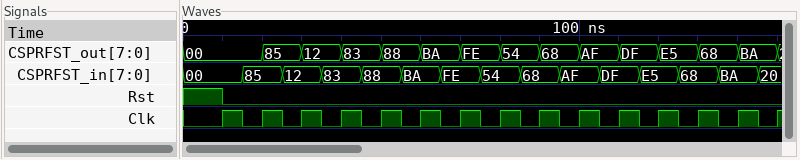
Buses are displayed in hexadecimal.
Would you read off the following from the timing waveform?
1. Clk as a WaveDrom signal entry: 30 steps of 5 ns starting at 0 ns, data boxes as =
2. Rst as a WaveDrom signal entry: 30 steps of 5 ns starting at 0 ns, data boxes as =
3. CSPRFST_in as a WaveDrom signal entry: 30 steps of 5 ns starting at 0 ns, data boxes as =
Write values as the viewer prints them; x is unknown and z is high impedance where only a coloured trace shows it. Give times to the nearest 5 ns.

{name: 'Clk', wave: '0.1010101010101010101010101010'}
{name: 'Rst', wave: '1.0...........................'}
{name: 'CSPRFST_in', wave: '=..=.=.=.=.=.=.=.=.=.=.=.=.=.=', data: '00 85 12 83 88 BA FE 54 68 AF DF E5 68 BA 20'}
